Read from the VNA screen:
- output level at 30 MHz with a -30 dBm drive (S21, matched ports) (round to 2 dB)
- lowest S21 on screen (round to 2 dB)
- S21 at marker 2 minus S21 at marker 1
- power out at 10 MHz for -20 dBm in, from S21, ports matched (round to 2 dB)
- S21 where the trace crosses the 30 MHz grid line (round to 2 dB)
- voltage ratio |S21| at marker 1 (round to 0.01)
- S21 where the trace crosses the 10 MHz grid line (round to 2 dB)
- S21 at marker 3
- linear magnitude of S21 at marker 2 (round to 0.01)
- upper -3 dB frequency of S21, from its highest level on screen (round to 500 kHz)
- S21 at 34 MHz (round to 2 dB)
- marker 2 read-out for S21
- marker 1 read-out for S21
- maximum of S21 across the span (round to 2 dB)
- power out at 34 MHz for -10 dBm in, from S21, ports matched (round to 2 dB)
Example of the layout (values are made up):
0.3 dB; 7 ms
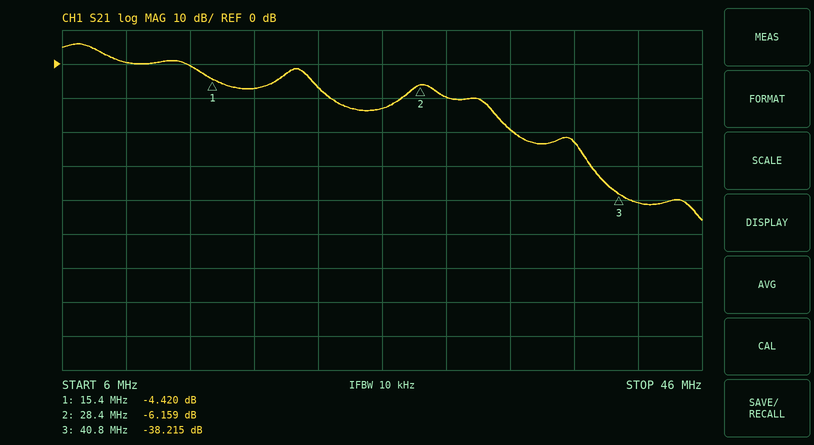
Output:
-40 dBm; -46 dB; -1.739 dB; -20 dBm; -10 dB; 0.60; 0 dB; -38.215 dB; 0.49; 8.5 MHz; -20 dB; -6.159 dB; -4.420 dB; 6 dB; -30 dBm
